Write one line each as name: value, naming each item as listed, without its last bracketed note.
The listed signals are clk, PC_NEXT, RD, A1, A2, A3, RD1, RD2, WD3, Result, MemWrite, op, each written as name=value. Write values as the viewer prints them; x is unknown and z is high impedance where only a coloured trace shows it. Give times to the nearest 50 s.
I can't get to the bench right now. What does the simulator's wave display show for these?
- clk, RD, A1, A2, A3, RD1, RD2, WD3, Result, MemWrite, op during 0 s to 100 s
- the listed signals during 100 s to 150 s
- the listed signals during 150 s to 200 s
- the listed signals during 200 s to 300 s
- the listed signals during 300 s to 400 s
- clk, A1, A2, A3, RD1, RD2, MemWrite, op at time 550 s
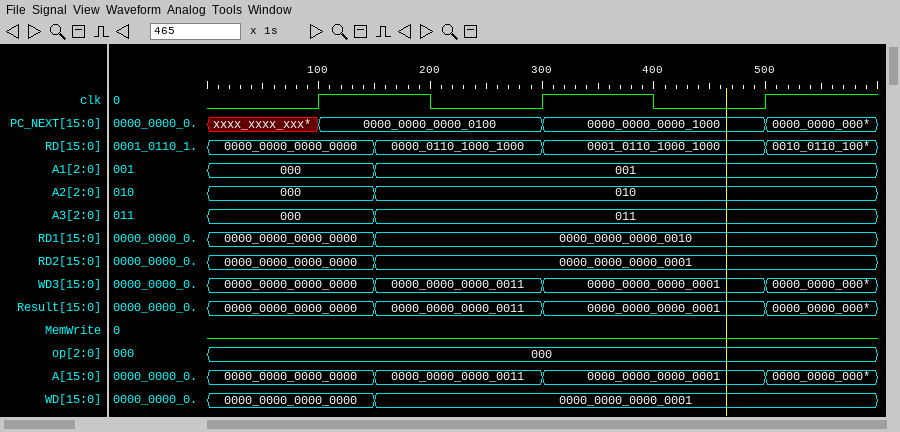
clk, RD, A1, A2, A3, RD1, RD2, WD3, Result, MemWrite, op during 0 s to 100 s: clk=0, RD=0000_0000_0000_0000, A1=000, A2=000, A3=000, RD1=0000_0000_0000_0000, RD2=0000_0000_0000_0000, WD3=0000_0000_0000_0000, Result=0000_0000_0000_0000, MemWrite=0, op=000
the listed signals during 100 s to 150 s: clk=1, PC_NEXT=0000_0000_0000_0100, RD=0000_0000_0000_0000, A1=000, A2=000, A3=000, RD1=0000_0000_0000_0000, RD2=0000_0000_0000_0000, WD3=0000_0000_0000_0000, Result=0000_0000_0000_0000, MemWrite=0, op=000
the listed signals during 150 s to 200 s: clk=1, PC_NEXT=0000_0000_0000_0100, RD=0000_0110_1000_1000, A1=001, A2=010, A3=011, RD1=0000_0000_0000_0010, RD2=0000_0000_0000_0001, WD3=0000_0000_0000_0011, Result=0000_0000_0000_0011, MemWrite=0, op=000
the listed signals during 200 s to 300 s: clk=0, PC_NEXT=0000_0000_0000_0100, RD=0000_0110_1000_1000, A1=001, A2=010, A3=011, RD1=0000_0000_0000_0010, RD2=0000_0000_0000_0001, WD3=0000_0000_0000_0011, Result=0000_0000_0000_0011, MemWrite=0, op=000
the listed signals during 300 s to 400 s: clk=1, PC_NEXT=0000_0000_0000_1000, RD=0001_0110_1000_1000, A1=001, A2=010, A3=011, RD1=0000_0000_0000_0010, RD2=0000_0000_0000_0001, WD3=0000_0000_0000_0001, Result=0000_0000_0000_0001, MemWrite=0, op=000
clk, A1, A2, A3, RD1, RD2, MemWrite, op at time 550 s: clk=1, A1=001, A2=010, A3=011, RD1=0000_0000_0000_0010, RD2=0000_0000_0000_0001, MemWrite=0, op=000
